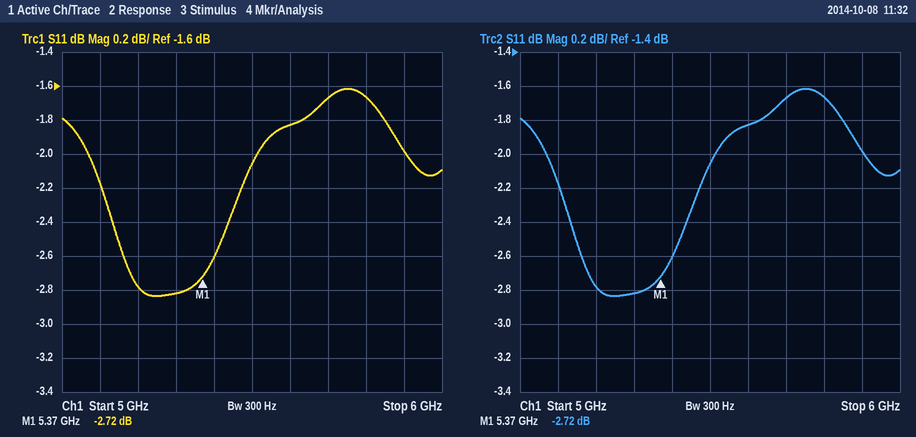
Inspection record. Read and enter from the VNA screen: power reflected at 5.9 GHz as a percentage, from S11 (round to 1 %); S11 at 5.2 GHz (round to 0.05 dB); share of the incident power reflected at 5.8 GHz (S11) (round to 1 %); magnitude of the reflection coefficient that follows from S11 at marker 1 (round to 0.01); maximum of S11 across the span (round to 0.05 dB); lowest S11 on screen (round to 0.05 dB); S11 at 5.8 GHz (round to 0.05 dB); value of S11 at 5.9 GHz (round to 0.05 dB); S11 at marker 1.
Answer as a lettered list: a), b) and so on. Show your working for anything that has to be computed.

a) 10^(-2/10) ≈ 63 %
b) -2.80 dB
c) 10^(-1.65/10) ≈ 68 %
d) 10^(-2.72/20) ≈ 0.73
e) -1.60 dB
f) -2.85 dB
g) -1.65 dB
h) -2.00 dB
i) -2.72 dB
